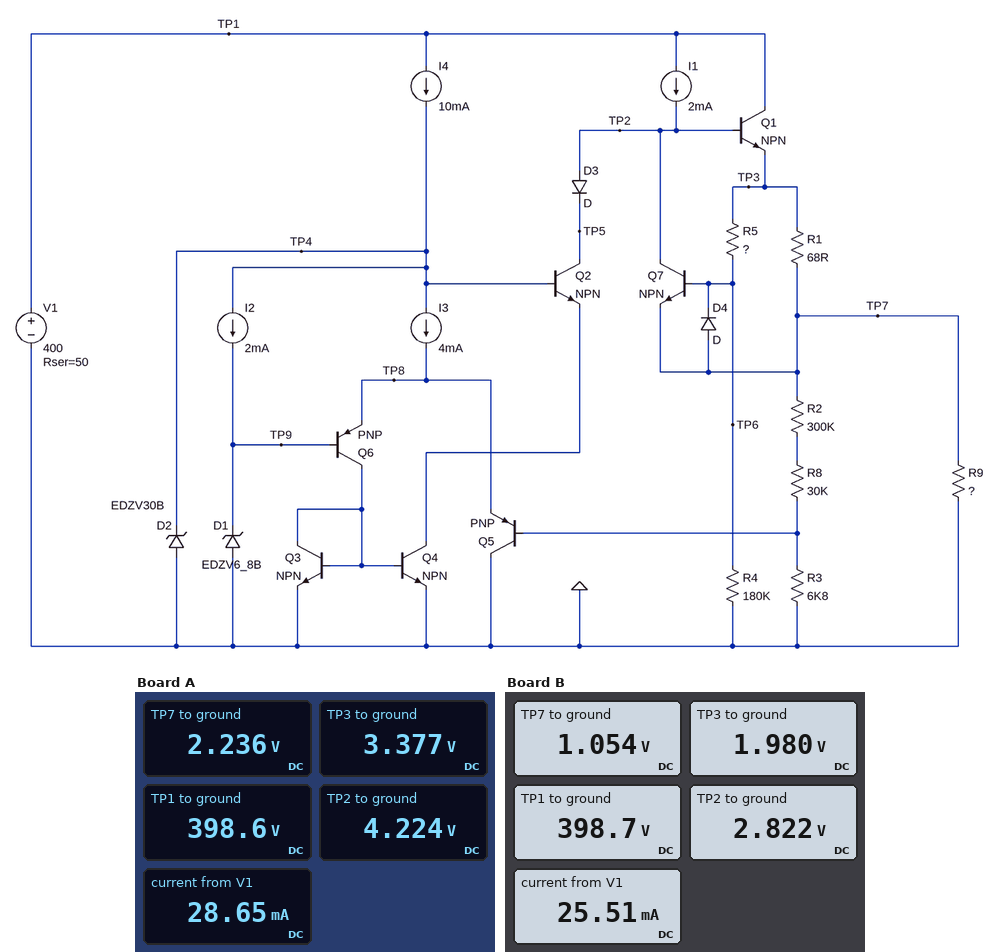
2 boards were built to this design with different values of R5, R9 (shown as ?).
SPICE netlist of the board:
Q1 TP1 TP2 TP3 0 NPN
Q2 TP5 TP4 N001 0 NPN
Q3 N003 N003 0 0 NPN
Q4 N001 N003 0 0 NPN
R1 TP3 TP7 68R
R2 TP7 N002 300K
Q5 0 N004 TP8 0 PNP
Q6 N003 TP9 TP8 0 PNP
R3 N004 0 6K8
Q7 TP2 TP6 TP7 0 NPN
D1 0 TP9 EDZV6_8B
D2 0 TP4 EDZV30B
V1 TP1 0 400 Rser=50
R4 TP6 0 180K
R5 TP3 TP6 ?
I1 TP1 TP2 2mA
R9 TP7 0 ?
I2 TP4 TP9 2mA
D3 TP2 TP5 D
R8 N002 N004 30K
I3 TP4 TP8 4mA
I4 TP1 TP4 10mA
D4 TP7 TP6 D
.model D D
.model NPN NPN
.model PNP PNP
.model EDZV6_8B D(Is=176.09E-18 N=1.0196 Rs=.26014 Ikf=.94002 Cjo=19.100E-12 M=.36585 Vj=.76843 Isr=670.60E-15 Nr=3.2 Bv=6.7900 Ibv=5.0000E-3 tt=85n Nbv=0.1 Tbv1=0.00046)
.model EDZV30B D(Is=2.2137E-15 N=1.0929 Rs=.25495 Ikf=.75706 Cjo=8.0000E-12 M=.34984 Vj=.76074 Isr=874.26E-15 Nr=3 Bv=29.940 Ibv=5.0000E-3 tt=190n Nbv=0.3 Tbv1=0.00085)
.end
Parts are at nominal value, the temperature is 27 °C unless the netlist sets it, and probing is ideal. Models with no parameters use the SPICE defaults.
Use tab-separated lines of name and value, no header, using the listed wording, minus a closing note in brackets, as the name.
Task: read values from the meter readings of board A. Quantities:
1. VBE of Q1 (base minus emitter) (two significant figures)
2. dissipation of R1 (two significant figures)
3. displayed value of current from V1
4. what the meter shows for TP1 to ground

VBE of Q1 (base minus emitter)	850 mV
dissipation of R1	19 mW
displayed value of current from V1	28.65 mA
what the meter shows for TP1 to ground	398.6 V
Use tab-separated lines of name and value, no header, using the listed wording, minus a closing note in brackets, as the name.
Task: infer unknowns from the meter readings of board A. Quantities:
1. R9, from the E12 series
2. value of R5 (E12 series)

R9, from the E12 series	120 Ω
value of R5	10 kΩ
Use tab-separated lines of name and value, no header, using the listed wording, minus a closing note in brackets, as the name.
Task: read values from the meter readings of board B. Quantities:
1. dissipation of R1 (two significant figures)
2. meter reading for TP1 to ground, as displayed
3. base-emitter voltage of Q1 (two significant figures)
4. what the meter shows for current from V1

dissipation of R1	13 mW
meter reading for TP1 to ground, as displayed	398.7 V
base-emitter voltage of Q1	840 mV
what the meter shows for current from V1	25.51 mA
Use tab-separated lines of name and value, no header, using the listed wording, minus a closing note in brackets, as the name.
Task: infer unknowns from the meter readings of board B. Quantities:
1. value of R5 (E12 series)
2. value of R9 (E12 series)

value of R5	4.7 kΩ
value of R9	68 Ω
